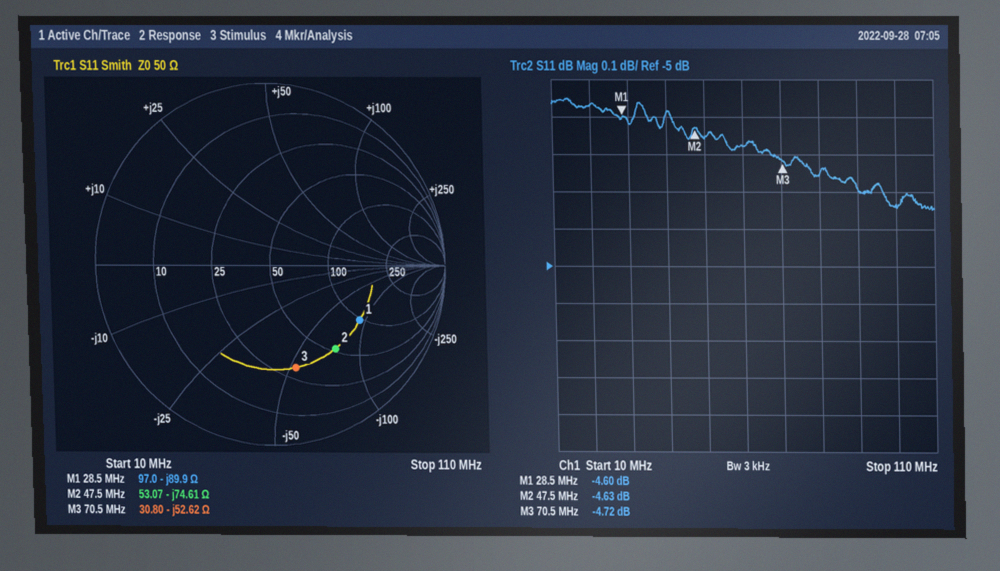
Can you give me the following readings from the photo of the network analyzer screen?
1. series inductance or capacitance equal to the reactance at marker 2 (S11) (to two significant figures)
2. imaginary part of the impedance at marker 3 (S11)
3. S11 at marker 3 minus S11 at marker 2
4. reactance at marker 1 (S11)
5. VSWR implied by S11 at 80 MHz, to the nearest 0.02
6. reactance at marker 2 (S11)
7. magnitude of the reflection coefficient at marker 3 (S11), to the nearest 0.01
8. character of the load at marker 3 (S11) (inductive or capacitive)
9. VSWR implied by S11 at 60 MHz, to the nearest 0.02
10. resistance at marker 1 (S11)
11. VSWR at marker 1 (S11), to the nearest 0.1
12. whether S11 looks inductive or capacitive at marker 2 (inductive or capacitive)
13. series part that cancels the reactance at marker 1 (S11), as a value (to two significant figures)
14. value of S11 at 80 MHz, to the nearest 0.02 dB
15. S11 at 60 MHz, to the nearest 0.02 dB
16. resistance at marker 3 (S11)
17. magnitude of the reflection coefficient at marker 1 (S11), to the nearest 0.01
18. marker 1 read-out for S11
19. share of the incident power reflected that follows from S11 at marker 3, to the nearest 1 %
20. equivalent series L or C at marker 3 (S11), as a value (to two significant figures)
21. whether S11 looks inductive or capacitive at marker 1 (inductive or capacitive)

45 pF
-52.62 Ω
-0.09 dB
-89.9 Ω
3.74
-74.61 Ω
0.58
capacitive
3.80
97.0 Ω
3.9
capacitive
500 nH
-4.76 dB
-4.68 dB
30.80 Ω
0.59
-4.60 dB
34 %
43 pF
capacitive
